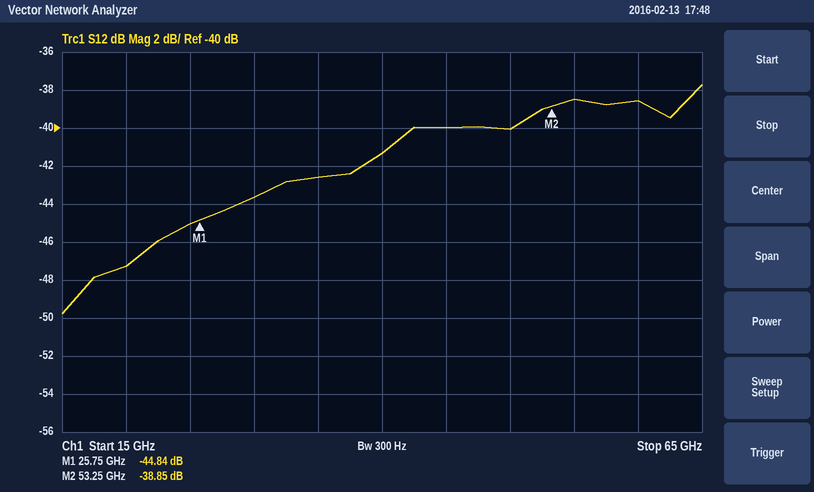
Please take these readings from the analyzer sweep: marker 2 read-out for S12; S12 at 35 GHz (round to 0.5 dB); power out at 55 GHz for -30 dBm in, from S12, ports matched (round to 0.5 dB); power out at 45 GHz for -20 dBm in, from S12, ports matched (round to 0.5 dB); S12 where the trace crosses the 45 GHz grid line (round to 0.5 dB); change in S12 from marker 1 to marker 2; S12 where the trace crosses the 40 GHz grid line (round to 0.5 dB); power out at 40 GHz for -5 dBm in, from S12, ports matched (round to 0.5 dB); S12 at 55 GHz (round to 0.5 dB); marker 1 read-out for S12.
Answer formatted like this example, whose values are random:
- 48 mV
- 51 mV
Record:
- -38.85 dB
- -42.5 dB
- -68.5 dBm
- -60.0 dBm
- -40.0 dB
- 5.99 dB
- -41.5 dB
- -46.5 dBm
- -38.5 dB
- -44.84 dB
